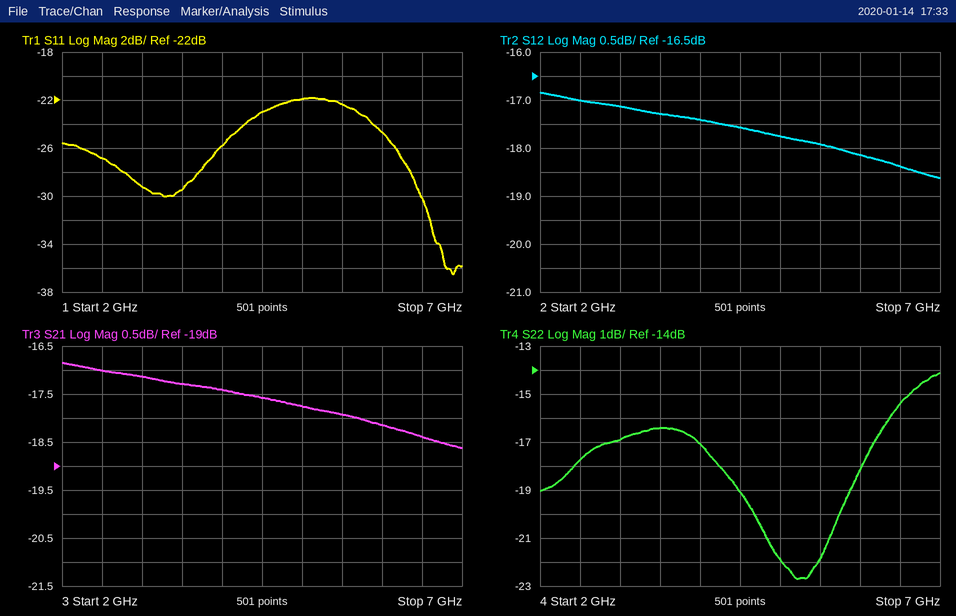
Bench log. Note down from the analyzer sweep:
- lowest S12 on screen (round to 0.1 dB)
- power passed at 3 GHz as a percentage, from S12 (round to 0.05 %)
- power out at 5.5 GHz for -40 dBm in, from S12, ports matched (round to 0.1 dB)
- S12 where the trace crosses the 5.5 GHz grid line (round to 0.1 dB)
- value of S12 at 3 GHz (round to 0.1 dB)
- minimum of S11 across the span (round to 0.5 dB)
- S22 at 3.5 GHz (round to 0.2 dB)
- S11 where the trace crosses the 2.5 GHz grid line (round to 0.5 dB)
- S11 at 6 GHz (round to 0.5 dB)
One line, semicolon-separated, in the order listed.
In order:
-18.6 dB; 1.95 %; -57.9 dBm; -17.9 dB; -17.1 dB; -36.5 dB; -16.4 dB; -27.0 dB; -24.5 dB
